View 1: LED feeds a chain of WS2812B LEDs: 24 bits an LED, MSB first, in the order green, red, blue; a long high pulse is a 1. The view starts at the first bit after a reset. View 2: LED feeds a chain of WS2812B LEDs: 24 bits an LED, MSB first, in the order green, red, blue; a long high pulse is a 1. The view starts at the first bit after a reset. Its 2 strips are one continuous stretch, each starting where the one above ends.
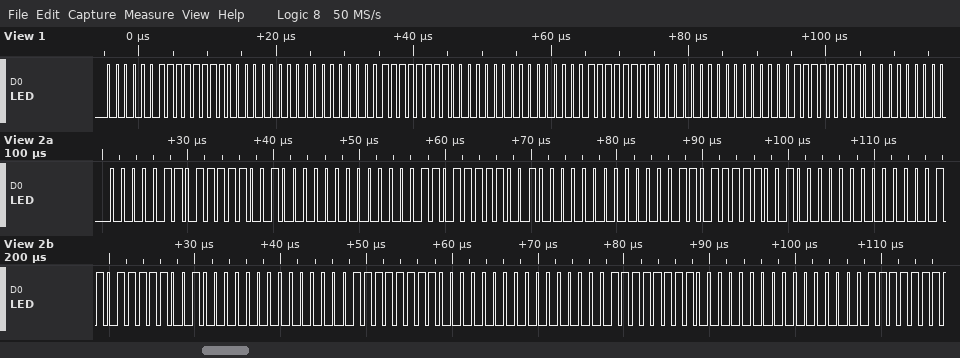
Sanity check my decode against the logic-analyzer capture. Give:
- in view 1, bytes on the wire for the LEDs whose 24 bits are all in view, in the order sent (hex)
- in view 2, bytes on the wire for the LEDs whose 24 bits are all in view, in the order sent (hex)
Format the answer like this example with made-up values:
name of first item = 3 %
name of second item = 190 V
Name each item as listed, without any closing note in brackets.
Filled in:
in view 1, bytes on the wire for the LEDs whose 24 bits are all in view, in the order sent = 03 FC 00 00 FF 00 00 FF 00 00 FF 00
in view 2, bytes on the wire for the LEDs whose 24 bits are all in view, in the order sent = 06 F9 00 06 F9 00 06 F9 00 06 F9 00 03 FC 00 03 FC 00
